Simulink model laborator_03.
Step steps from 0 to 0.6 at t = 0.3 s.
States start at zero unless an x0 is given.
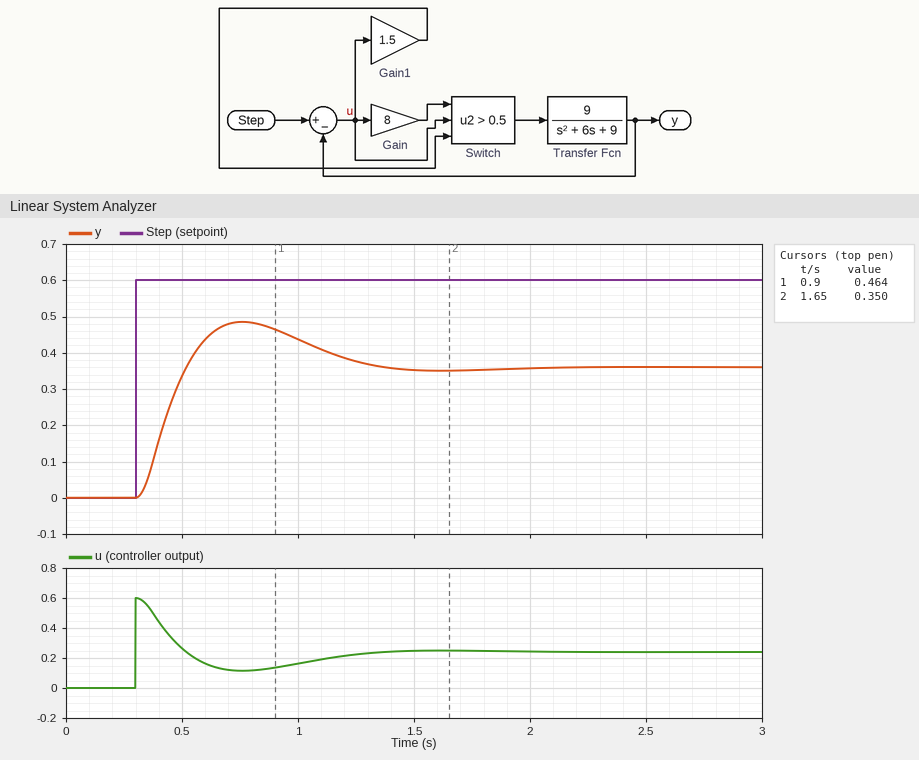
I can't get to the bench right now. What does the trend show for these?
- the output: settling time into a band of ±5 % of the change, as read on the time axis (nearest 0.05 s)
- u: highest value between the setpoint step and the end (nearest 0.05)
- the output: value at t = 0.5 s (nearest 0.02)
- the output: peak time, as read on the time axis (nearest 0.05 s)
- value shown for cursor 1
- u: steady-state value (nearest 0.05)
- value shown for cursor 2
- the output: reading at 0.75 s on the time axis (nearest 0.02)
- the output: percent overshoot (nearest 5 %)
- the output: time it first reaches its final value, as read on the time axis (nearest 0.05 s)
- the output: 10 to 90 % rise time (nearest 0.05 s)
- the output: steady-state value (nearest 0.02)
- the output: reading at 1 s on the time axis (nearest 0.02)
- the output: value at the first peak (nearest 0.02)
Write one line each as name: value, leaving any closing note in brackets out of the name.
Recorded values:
the output: settling time into a band of ±5 % of the change, as read on the time axis: 1.25 s
u: highest value between the setpoint step and the end: 0.60
the output: value at t = 0.5 s: 0.34
the output: peak time, as read on the time axis: 0.75 s
value shown for cursor 1: 0.464
u: steady-state value: 0.25
value shown for cursor 2: 0.350
the output: reading at 0.75 s on the time axis: 0.48
the output: percent overshoot: 35 %
the output: time it first reaches its final value, as read on the time axis: 0.50 s
the output: 10 to 90 % rise time: 0.15 s
the output: steady-state value: 0.36
the output: reading at 1 s on the time axis: 0.44
the output: value at the first peak: 0.48
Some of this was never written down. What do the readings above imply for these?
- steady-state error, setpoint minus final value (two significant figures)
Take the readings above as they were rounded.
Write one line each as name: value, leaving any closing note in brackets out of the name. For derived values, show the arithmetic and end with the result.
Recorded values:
steady-state error, setpoint minus final value: 0.6 - 0.36 = 0.24
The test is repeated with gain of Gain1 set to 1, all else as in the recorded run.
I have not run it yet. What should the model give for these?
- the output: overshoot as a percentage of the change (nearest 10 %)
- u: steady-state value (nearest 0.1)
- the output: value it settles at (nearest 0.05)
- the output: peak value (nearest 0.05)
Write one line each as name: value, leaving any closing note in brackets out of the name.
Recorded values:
the output: overshoot as a percentage of the change: 50 %
u: steady-state value: 0.3
the output: value it settles at: 0.30
the output: peak value: 0.45
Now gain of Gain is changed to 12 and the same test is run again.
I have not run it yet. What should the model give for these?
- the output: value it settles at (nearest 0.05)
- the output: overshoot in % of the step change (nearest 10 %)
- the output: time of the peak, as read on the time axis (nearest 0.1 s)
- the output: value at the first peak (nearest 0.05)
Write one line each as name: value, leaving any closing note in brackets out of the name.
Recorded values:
the output: value it settles at: 0.35
the output: overshoot in % of the step change: 50 %
the output: time of the peak, as read on the time axis: 0.7 s
the output: value at the first peak: 0.55
